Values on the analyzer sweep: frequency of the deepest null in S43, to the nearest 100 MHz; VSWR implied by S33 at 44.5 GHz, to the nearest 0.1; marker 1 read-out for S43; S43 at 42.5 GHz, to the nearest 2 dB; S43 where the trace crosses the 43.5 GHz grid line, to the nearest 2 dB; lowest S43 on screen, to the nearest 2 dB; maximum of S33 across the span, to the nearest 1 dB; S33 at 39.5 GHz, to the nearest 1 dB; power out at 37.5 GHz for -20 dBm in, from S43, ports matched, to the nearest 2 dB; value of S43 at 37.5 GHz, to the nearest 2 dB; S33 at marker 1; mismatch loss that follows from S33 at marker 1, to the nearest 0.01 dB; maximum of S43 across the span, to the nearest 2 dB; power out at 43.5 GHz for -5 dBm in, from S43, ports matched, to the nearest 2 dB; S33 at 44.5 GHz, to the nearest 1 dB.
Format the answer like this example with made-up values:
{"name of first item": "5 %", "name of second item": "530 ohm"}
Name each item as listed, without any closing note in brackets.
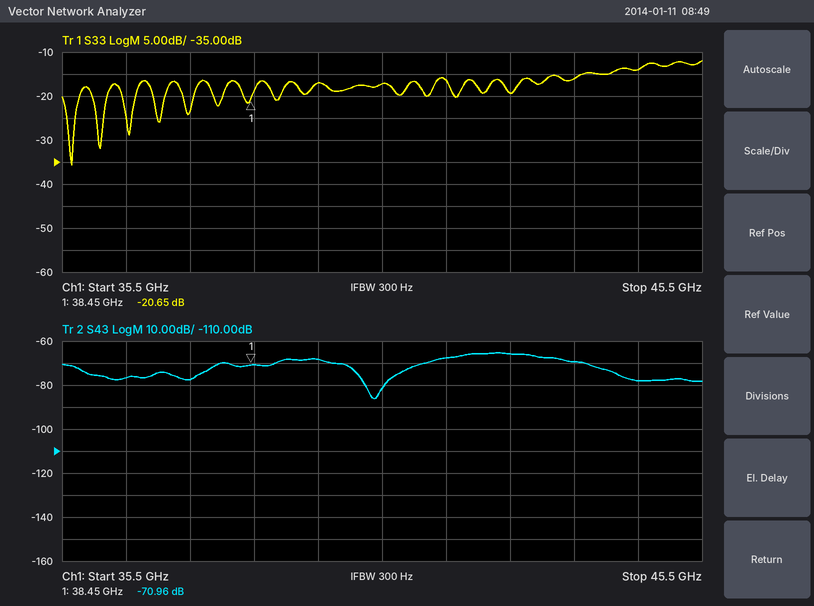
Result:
{"frequency of the deepest null in S43, to the nearest 100 MHz": "40.4 GHz", "VSWR implied by S33 at 44.5 GHz, to the nearest 0.1": "1.5", "marker 1 read-out for S43": "-70.96 dB", "S43 at 42.5 GHz, to the nearest 2 dB": "-66 dB", "S43 where the trace crosses the 43.5 GHz grid line, to the nearest 2 dB": "-70 dB", "lowest S43 on screen, to the nearest 2 dB": "-86 dB", "maximum of S33 across the span, to the nearest 1 dB": "-12 dB", "S33 at 39.5 GHz, to the nearest 1 dB": "-17 dB", "power out at 37.5 GHz for -20 dBm in, from S43, ports matched, to the nearest 2 dB": "-98 dBm", "value of S43 at 37.5 GHz, to the nearest 2 dB": "-78 dB", "S33 at marker 1": "-20.65 dB", "mismatch loss that follows from S33 at marker 1, to the nearest 0.01 dB": "0.04 dB", "maximum of S43 across the span, to the nearest 2 dB": "-66 dB", "power out at 43.5 GHz for -5 dBm in, from S43, ports matched, to the nearest 2 dB": "-74 dBm", "S33 at 44.5 GHz, to the nearest 1 dB": "-14 dB"}
